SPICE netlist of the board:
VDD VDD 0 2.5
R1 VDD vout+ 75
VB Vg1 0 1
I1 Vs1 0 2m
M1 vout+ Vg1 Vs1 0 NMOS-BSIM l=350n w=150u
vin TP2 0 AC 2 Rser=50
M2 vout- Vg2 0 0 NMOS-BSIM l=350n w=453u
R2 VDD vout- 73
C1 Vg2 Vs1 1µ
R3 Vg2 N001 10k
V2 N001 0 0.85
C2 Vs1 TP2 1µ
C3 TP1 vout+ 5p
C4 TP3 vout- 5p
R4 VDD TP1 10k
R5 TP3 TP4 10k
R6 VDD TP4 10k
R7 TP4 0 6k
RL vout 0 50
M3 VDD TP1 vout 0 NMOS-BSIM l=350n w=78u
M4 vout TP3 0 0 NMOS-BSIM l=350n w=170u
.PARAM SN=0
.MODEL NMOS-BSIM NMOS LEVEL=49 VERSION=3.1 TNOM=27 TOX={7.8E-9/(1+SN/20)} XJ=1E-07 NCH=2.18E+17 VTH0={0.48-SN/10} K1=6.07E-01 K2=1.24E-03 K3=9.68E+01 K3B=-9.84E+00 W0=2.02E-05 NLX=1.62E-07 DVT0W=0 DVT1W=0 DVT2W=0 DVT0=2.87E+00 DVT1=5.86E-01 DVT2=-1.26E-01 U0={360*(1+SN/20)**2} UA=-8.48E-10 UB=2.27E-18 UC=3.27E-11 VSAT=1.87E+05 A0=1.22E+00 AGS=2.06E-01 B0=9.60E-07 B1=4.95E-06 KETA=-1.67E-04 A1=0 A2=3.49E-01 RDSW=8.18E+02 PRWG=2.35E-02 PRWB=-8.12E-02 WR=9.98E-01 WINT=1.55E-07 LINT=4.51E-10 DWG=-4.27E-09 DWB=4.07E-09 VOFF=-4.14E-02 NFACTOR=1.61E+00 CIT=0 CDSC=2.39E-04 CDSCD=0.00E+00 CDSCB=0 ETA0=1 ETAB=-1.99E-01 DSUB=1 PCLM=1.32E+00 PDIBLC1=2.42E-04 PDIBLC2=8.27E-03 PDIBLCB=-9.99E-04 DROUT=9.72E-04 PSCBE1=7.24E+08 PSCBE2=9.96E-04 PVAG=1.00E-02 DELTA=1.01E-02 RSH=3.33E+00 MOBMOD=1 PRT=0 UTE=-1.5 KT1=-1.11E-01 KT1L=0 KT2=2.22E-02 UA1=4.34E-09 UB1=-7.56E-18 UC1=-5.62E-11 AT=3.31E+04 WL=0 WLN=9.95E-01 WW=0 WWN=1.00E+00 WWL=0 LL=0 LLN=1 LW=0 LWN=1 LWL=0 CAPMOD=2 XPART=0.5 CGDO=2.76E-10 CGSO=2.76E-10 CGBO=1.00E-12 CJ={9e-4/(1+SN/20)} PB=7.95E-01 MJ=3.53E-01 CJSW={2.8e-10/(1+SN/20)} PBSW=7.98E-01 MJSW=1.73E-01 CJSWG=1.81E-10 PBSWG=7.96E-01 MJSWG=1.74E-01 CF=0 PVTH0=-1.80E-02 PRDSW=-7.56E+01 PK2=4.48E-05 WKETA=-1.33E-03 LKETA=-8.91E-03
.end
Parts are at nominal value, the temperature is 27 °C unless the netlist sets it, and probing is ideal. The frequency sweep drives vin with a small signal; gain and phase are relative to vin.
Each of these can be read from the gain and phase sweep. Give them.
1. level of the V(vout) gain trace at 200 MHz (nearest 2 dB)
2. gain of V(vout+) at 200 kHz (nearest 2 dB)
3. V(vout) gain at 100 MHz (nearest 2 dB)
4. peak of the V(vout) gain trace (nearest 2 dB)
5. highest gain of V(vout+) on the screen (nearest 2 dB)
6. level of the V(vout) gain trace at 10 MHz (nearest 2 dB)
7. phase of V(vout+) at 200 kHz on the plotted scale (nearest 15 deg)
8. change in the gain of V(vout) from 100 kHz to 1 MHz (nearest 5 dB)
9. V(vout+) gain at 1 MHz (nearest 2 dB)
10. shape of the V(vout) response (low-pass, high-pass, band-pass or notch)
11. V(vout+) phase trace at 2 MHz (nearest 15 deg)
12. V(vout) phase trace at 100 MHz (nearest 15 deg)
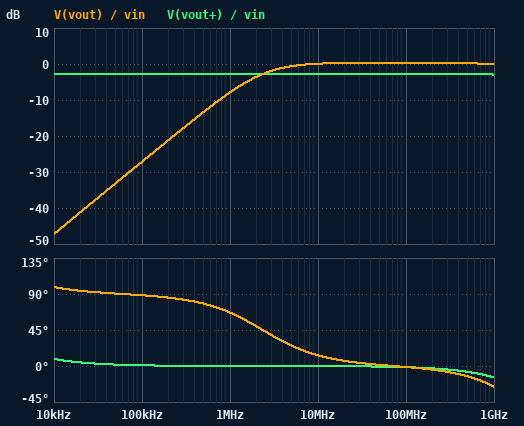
0 dB
-2 dB
0 dB
0 dB
-2 dB
0 dB
0 deg
20 dB
-2 dB
high-pass
0 deg
0 deg
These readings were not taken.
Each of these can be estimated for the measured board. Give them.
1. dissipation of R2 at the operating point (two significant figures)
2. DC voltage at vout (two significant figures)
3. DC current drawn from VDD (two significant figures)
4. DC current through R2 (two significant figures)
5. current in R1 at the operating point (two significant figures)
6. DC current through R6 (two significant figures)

4.6 mW
530 mV
25 mA
8.0 mA
2.0 mA
160 µA
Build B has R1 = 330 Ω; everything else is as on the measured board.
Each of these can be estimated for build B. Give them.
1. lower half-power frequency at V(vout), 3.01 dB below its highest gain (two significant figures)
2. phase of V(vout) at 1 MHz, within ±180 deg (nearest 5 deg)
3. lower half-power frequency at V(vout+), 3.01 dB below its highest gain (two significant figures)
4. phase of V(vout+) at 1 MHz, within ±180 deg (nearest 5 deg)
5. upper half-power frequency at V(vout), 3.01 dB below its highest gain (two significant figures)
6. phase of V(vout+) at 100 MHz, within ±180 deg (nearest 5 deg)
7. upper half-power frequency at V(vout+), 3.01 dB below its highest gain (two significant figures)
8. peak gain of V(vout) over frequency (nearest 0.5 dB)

2.7 MHz
70 deg
1.5 kHz
0 deg
2.6 GHz
-5 deg
2.5 GHz
5.5 dB
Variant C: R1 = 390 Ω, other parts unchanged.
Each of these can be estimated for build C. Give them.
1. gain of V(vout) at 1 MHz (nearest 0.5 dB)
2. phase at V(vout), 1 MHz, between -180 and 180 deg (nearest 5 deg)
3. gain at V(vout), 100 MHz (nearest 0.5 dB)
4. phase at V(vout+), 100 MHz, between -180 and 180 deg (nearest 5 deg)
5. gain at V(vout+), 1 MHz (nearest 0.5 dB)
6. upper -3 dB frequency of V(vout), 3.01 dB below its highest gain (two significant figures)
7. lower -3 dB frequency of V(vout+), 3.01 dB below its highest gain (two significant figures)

-2.5 dB
70 deg
6.5 dB
-5 deg
11.0 dB
2.4 GHz
1.5 kHz
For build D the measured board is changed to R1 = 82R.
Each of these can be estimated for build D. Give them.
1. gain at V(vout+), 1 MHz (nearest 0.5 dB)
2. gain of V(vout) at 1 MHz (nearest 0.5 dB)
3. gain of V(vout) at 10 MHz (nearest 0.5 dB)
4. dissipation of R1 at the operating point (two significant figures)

-2.0 dB
-7.5 dB
0.5 dB
330 µW
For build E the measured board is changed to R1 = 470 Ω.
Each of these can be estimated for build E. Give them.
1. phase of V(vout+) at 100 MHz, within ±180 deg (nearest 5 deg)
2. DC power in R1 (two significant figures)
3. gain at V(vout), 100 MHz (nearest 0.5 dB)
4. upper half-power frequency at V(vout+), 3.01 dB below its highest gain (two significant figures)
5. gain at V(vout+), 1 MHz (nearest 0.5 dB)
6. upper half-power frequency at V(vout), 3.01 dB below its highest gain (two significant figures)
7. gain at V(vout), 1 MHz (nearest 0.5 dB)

-5 deg
1.9 mW
7.5 dB
1.9 GHz
12.5 dB
2.2 GHz
-1.5 dB
